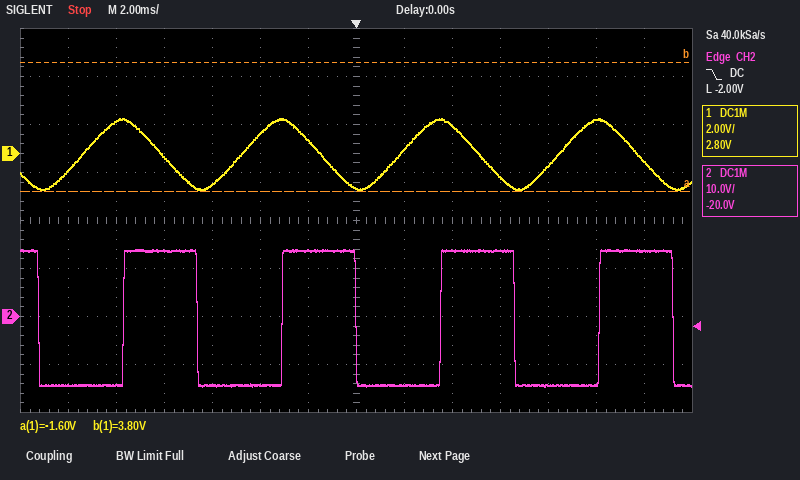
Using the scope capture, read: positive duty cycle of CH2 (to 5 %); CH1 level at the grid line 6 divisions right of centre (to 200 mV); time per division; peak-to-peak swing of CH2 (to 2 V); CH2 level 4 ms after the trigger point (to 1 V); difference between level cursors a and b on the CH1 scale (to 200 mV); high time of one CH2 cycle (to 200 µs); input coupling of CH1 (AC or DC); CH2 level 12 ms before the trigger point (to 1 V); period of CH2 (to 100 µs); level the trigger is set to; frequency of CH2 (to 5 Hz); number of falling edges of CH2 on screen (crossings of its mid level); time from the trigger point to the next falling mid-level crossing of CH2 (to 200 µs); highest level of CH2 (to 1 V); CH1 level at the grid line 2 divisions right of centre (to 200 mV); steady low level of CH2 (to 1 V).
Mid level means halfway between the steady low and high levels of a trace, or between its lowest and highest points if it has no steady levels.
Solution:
45 %
-400 mV
2 ms
28 V
14 V
5.4 V
3.0 ms
DC
-14 V
6.6 ms
-2.00 V
150 Hz
5
6.6 ms
14 V
1.2 V
-14 V
